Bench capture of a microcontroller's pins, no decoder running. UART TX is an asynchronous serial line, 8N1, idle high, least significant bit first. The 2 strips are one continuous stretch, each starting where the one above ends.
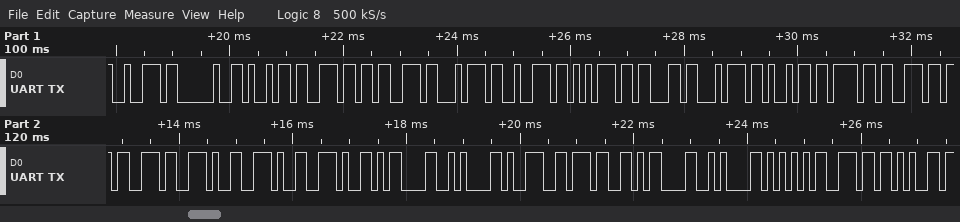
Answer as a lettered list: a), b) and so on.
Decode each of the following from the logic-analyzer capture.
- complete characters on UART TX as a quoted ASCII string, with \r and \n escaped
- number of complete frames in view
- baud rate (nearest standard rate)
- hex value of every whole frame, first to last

a) "r instructions...\r\n97\r\nUne"
b) 26
c) 9600 baud
d) 72 20 69 6E 73 74 72 75 63 74 69 6F 6E 73 2E 2E 2E 0D 0A 39 37 0D 0A 55 6E 65
